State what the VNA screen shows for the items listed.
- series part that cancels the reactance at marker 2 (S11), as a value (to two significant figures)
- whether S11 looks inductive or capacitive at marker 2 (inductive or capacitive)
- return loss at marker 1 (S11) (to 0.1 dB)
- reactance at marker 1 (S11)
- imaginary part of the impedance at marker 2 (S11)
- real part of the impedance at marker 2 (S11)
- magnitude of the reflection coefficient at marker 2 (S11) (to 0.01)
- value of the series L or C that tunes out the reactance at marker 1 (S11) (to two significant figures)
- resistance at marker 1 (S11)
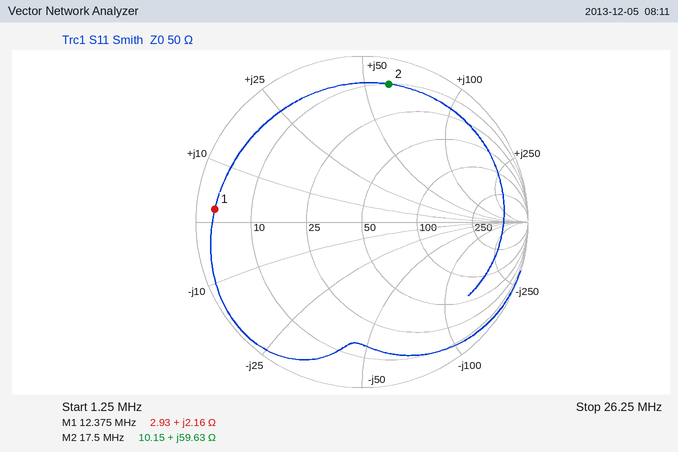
150 pF
inductive
1.0 dB
+2.16 Ω
+59.63 Ω
10.15 Ω
0.85
6.0 nF
2.93 Ω
